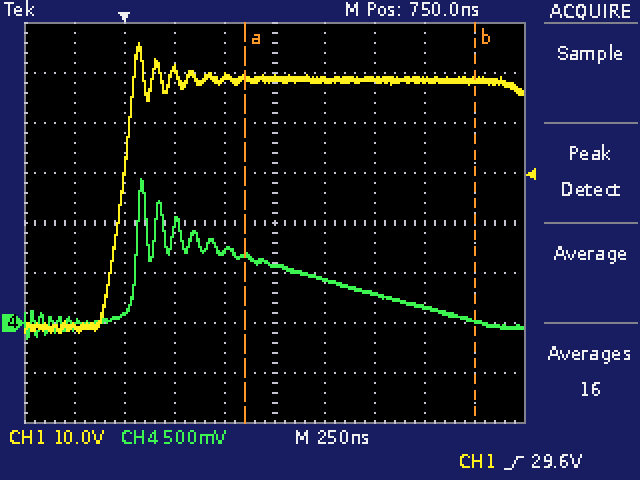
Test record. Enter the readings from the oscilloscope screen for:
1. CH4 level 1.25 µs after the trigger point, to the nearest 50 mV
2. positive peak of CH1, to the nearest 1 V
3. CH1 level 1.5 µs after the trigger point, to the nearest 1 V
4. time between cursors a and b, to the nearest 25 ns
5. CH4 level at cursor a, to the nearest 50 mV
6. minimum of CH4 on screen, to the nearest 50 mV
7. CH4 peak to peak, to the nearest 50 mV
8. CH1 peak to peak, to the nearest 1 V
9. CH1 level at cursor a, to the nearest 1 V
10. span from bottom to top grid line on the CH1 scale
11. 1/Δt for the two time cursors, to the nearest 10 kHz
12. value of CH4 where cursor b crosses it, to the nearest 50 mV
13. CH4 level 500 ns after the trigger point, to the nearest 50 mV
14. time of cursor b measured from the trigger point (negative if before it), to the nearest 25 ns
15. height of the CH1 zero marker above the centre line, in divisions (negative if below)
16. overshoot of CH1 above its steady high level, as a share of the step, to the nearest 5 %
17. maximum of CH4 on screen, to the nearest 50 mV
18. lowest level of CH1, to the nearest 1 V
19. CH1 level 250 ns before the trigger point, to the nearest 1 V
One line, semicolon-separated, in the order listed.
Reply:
300 mV; 56 V; 49 V; 1.150 µs; 650 mV; -150 mV; 1.60 V; 58 V; 49 V; 80 V; 870 kHz; 0 mV; 700 mV; +1.750 µs; -2.0 div; 15 %; 1.45 V; -2 V; -1 V
